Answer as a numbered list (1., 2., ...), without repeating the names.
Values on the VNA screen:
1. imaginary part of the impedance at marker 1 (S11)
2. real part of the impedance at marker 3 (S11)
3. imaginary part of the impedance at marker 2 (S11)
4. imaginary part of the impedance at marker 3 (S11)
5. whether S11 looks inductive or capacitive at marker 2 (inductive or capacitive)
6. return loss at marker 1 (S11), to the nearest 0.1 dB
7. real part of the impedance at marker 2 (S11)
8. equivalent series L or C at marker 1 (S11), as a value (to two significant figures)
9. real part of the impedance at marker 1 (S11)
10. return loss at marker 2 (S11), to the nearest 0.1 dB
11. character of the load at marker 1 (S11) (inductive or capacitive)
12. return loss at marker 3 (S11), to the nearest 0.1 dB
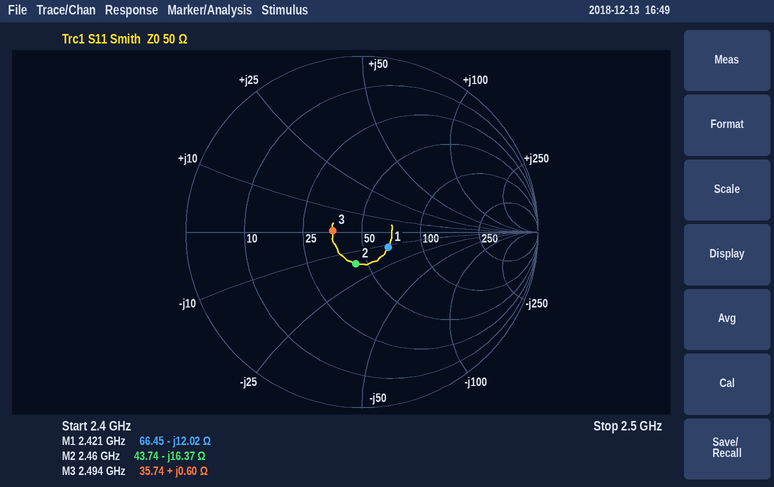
1. -12.02 Ω
2. 35.74 Ω
3. -16.37 Ω
4. +0.60 Ω
5. capacitive
6. 15.2 dB
7. 43.74 Ω
8. 5.5 pF
9. 66.45 Ω
10. 14.7 dB
11. capacitive
12. 15.6 dB
